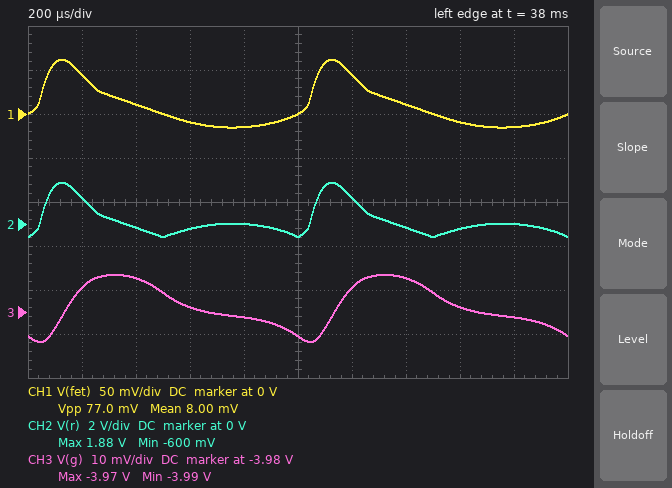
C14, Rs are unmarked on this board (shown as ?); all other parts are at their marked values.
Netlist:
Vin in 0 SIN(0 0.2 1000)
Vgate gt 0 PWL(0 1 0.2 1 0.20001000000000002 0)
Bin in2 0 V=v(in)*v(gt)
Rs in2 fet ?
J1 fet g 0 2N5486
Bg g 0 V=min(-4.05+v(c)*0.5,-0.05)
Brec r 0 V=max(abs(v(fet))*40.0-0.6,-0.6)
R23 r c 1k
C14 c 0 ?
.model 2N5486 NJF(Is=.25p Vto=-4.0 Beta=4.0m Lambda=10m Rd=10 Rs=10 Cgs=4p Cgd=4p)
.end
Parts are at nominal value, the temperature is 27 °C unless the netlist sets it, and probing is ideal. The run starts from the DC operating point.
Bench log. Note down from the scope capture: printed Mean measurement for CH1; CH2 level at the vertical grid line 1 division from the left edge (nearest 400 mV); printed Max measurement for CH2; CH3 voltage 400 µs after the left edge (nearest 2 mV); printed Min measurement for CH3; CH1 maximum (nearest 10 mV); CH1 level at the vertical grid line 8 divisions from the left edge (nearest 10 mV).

8.00 mV
1.2 V
1.88 V
-3.972 V
-3.99 V
60 mV
-10 mV
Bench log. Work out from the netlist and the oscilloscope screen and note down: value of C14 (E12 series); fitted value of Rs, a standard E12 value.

8.2 µF
56 kΩ
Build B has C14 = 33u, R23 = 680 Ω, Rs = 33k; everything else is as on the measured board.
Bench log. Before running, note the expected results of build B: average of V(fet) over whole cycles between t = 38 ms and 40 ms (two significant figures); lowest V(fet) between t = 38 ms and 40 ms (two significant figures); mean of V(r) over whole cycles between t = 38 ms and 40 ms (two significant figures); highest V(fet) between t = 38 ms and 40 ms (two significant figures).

7.7 mV
-17 mV
160 mV
61 mV
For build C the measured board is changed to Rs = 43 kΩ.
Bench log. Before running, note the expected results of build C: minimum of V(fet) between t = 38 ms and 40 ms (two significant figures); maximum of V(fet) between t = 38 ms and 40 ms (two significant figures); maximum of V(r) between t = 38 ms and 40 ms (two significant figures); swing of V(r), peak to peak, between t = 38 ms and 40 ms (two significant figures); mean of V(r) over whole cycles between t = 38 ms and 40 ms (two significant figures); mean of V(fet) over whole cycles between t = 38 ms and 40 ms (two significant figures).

-17 mV
60 mV
1.8 V
2.4 V
150 mV
7.7 mV
